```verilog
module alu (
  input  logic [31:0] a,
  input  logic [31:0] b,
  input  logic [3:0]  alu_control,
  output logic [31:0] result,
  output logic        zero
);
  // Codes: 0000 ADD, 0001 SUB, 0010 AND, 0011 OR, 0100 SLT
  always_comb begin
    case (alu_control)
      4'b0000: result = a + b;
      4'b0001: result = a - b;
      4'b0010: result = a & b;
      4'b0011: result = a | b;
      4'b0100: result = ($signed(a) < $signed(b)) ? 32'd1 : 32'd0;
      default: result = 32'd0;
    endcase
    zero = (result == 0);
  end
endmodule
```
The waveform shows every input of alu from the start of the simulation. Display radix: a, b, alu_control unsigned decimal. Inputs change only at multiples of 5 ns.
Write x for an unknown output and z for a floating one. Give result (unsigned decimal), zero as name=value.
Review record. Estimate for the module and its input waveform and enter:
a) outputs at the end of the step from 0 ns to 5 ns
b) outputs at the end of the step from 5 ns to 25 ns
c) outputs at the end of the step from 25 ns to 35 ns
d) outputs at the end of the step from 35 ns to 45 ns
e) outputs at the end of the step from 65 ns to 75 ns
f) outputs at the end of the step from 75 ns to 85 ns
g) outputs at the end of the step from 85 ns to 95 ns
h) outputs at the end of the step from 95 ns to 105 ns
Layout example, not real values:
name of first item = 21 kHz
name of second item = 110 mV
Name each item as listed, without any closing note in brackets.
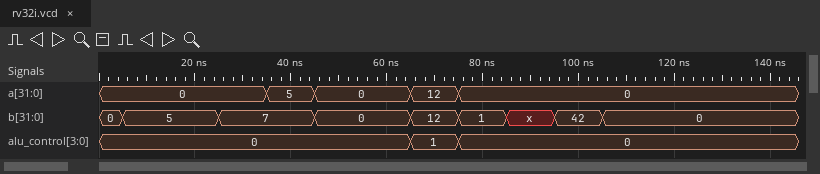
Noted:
outputs at the end of the step from 0 ns to 5 ns = result=0, zero=1
outputs at the end of the step from 5 ns to 25 ns = result=5, zero=0
outputs at the end of the step from 25 ns to 35 ns = result=7, zero=0
outputs at the end of the step from 35 ns to 45 ns = result=12, zero=0
outputs at the end of the step from 65 ns to 75 ns = result=0, zero=1
outputs at the end of the step from 75 ns to 85 ns = result=1, zero=0
outputs at the end of the step from 85 ns to 95 ns = result=x, zero=x
outputs at the end of the step from 95 ns to 105 ns = result=42, zero=0
